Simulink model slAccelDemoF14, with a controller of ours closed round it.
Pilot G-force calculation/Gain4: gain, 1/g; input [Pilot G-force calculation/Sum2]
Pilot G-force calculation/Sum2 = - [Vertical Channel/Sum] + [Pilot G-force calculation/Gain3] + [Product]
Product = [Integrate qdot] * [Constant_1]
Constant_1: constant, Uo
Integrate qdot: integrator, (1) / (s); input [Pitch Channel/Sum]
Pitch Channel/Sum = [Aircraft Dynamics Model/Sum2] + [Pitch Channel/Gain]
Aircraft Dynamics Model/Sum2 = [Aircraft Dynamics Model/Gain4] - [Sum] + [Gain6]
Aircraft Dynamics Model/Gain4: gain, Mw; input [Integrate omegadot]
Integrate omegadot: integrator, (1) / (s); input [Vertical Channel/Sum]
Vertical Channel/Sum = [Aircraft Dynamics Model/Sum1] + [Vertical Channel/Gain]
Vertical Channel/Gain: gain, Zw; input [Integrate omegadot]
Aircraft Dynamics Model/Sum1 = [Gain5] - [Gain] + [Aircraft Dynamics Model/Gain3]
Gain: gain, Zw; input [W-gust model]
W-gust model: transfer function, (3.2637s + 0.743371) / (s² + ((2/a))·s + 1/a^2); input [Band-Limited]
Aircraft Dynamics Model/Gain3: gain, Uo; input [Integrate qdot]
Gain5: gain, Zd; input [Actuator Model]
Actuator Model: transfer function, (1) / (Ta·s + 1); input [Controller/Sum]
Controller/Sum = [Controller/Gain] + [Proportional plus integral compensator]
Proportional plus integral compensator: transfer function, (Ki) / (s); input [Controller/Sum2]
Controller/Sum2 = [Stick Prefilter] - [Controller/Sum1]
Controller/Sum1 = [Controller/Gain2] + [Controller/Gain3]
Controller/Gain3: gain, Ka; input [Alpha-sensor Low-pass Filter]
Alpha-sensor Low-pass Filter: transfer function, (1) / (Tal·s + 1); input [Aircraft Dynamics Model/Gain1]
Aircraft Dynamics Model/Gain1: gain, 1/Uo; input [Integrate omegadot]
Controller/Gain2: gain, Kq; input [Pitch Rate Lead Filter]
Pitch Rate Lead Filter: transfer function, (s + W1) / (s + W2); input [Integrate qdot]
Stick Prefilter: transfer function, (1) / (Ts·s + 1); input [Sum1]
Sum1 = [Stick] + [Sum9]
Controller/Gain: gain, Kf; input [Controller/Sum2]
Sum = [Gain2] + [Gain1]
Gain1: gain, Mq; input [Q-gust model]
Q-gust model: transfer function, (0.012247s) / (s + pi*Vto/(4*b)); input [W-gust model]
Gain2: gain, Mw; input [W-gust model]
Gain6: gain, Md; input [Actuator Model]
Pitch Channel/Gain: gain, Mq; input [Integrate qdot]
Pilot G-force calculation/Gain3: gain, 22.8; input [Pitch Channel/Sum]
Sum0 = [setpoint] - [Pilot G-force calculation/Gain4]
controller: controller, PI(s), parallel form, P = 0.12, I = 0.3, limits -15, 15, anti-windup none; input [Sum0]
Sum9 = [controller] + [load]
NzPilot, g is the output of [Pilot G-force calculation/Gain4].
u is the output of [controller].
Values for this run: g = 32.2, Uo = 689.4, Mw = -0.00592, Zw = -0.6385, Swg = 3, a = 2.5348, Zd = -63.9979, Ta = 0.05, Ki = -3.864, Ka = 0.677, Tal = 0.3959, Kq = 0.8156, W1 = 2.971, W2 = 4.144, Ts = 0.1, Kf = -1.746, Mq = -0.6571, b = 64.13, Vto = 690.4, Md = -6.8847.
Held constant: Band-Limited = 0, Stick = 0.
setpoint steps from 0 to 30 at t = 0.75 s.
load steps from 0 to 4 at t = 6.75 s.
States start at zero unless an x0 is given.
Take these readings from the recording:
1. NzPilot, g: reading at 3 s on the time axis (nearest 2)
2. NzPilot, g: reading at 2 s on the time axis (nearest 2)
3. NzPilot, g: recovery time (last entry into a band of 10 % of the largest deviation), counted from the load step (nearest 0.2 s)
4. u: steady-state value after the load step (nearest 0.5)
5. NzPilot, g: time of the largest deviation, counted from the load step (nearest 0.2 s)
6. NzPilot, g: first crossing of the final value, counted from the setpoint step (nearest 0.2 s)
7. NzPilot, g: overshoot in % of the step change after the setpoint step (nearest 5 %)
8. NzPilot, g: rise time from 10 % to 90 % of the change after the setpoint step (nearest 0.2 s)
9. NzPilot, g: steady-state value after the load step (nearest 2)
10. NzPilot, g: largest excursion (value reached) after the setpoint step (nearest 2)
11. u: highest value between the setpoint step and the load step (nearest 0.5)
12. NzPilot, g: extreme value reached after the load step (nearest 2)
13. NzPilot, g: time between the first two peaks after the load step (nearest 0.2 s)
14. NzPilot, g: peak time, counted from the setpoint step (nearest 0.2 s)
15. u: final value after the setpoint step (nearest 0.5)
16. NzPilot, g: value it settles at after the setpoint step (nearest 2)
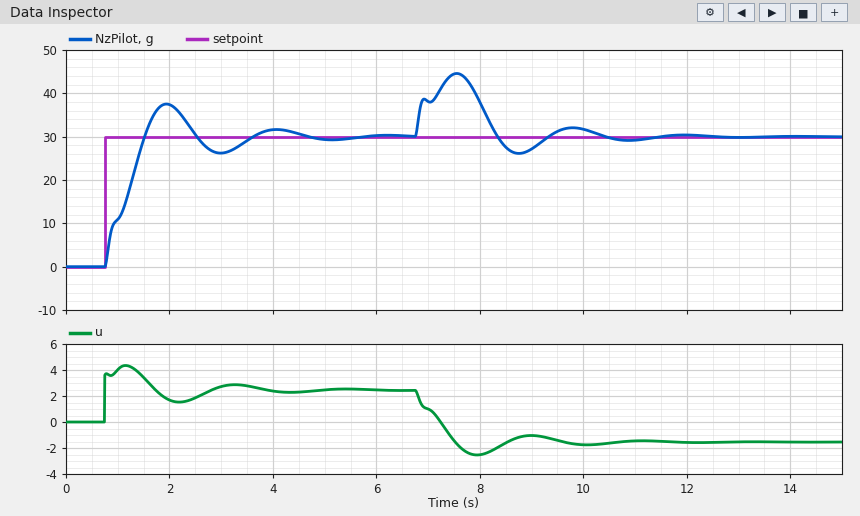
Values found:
26
38
3.4 s
-1.5
0.8 s
0.8 s
25 %
0.6 s
30
38
4.5
44
2.2 s
1.2 s
2.5
30
